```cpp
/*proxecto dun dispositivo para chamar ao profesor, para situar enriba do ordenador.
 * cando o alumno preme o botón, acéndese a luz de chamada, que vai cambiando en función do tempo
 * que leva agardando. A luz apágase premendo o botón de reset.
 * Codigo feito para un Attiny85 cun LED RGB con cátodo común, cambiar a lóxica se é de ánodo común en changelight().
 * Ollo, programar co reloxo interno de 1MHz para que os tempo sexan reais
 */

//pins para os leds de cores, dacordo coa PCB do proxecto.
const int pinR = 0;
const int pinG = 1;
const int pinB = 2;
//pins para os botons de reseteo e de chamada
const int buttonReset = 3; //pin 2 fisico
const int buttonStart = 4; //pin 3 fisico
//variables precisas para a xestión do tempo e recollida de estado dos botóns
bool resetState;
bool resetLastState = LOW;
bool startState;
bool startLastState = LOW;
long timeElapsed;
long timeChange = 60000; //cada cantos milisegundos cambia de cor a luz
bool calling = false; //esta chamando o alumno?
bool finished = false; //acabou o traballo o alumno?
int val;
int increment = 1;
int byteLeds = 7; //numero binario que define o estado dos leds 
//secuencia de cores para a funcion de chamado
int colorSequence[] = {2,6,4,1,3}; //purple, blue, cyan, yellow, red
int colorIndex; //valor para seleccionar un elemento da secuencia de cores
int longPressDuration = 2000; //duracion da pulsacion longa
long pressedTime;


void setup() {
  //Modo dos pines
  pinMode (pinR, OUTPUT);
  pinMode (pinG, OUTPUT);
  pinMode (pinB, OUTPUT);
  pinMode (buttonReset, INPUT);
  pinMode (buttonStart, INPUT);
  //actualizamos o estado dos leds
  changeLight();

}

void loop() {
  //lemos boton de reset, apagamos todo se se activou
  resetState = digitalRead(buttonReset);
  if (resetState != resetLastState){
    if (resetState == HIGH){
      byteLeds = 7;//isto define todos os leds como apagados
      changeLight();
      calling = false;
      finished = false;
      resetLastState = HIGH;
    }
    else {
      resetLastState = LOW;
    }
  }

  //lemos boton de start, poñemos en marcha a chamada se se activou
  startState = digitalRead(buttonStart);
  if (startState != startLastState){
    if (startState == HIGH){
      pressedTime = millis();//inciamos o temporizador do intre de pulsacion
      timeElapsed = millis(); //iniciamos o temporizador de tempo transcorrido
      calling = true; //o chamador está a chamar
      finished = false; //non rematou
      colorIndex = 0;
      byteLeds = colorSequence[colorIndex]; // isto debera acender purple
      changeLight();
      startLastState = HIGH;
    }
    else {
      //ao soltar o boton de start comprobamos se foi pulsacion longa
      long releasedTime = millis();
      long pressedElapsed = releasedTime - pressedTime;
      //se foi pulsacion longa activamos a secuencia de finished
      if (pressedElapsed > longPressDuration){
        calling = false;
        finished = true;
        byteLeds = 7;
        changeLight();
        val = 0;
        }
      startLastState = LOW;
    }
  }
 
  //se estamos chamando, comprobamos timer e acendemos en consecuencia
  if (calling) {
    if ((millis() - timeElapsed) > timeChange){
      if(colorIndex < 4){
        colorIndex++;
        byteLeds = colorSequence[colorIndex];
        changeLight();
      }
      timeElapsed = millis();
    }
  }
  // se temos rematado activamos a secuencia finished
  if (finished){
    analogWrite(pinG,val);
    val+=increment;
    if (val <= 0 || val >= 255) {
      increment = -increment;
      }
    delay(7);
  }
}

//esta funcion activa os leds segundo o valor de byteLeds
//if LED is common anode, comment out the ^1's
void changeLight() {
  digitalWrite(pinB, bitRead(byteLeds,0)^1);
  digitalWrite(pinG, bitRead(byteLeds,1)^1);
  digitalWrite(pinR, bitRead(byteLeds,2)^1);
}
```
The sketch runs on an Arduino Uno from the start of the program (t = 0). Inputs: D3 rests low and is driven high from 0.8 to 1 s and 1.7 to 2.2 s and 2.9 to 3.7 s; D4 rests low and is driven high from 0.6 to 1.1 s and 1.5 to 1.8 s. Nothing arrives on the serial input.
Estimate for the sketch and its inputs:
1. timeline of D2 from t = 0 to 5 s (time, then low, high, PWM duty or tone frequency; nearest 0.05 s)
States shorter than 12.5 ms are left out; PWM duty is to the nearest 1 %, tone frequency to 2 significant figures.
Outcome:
0 s low; 0.6 s high; 0.8 s low; 1.5 s high; 1.7 s low
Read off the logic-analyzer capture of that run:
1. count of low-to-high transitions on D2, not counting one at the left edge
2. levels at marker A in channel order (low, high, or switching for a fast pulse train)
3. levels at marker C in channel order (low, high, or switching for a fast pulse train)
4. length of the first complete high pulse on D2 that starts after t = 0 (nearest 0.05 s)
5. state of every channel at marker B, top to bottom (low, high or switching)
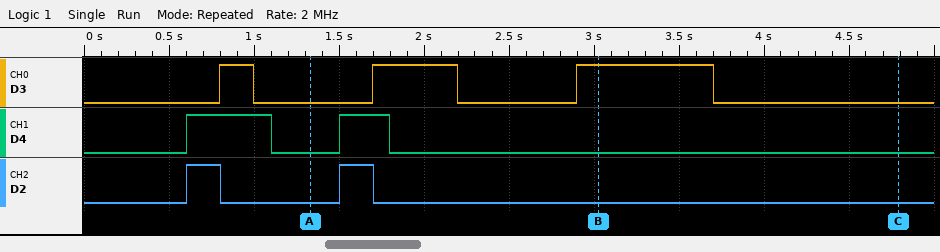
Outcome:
2
D3 low, D4 low, D2 low
D3 low, D4 low, D2 low
0.20 s
D3 high, D4 low, D2 low
